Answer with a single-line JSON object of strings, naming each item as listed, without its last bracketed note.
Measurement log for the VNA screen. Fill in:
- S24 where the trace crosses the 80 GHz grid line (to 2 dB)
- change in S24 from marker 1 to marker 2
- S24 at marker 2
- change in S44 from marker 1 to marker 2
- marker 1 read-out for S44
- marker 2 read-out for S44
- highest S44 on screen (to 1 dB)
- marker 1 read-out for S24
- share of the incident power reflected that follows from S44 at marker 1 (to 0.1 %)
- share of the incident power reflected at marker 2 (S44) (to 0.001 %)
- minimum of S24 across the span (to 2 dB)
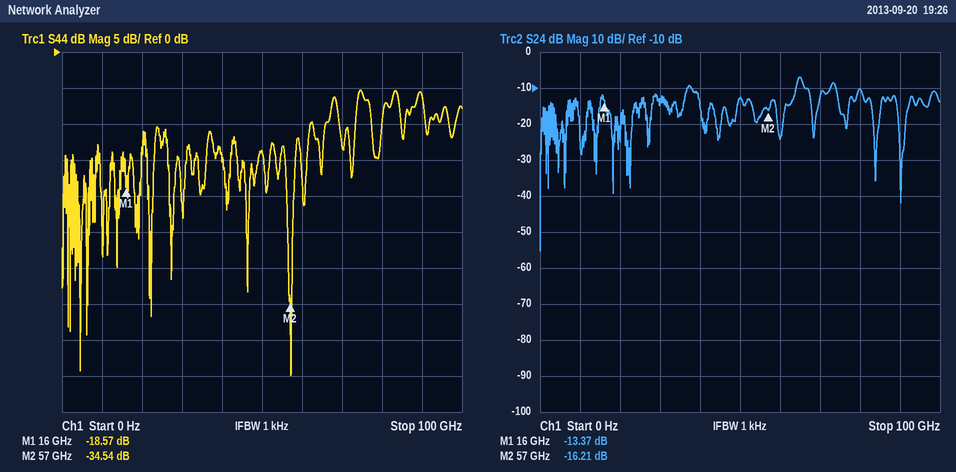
{"S24 where the trace crosses the 80 GHz grid line": "-10 dB", "change in S24 from marker 1 to marker 2": "-2.84 dB", "S24 at marker 2": "-16.21 dB", "change in S44 from marker 1 to marker 2": "-15.97 dB", "marker 1 read-out for S44": "-18.57 dB", "marker 2 read-out for S44": "-34.54 dB", "highest S44 on screen": "-5 dB", "marker 1 read-out for S24": "-13.37 dB", "share of the incident power reflected that follows from S44 at marker 1": "1.4 %", "share of the incident power reflected at marker 2 (S44)": "0.035 %", "minimum of S24 across the span": "-56 dB"}
